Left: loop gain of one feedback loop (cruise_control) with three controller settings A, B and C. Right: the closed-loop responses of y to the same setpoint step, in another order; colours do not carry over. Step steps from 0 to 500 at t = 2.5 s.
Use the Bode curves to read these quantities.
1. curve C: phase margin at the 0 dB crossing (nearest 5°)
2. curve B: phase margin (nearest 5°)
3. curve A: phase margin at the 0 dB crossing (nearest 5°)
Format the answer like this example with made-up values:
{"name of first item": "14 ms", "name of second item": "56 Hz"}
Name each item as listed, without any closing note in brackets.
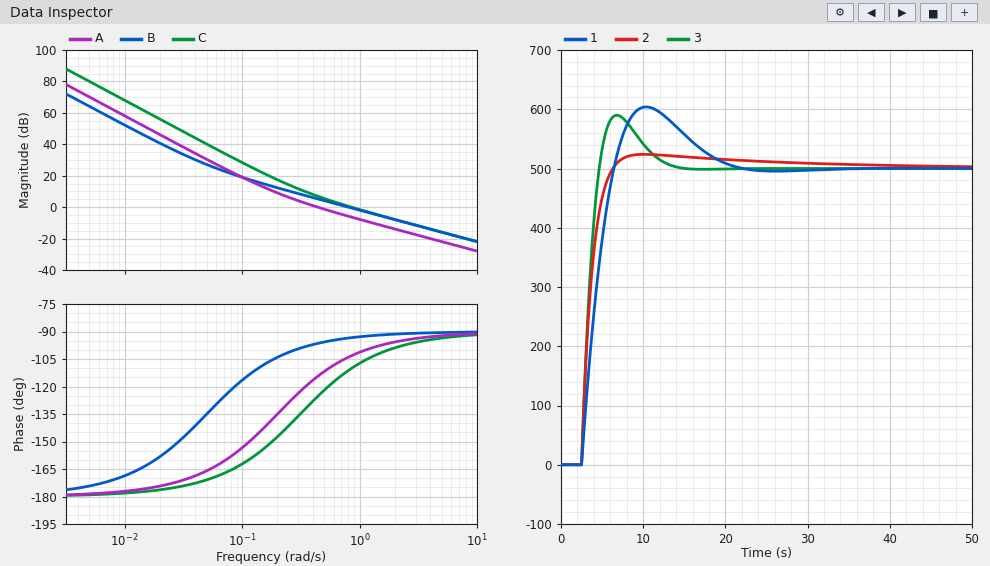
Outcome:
{"curve C: phase margin at the 0 dB crossing": "70°", "curve B: phase margin": "85°", "curve A: phase margin at the 0 dB crossing": "65°"}
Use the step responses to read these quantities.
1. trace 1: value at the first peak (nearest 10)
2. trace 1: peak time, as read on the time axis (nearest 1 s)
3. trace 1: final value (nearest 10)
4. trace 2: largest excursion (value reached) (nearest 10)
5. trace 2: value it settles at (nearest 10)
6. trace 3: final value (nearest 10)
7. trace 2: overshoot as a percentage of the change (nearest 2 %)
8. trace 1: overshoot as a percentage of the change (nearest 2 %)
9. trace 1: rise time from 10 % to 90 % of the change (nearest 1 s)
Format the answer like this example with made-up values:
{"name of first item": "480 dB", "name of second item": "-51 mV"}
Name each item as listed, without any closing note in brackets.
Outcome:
{"trace 1: value at the first peak": "600", "trace 1: peak time, as read on the time axis": "10 s", "trace 1: final value": "500", "trace 2: largest excursion (value reached)": "520", "trace 2: value it settles at": "500", "trace 3: final value": "500", "trace 2: overshoot as a percentage of the change": "4 %", "trace 1: overshoot as a percentage of the change": "20 %", "trace 1: rise time from 10 % to 90 % of the change": "3 s"}
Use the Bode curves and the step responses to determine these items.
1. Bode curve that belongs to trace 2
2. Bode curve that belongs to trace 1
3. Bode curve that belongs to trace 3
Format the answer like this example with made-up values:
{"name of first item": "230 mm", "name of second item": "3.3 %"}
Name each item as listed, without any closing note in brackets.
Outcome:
{"Bode curve that belongs to trace 2": "B", "Bode curve that belongs to trace 1": "A", "Bode curve that belongs to trace 3": "C"}
